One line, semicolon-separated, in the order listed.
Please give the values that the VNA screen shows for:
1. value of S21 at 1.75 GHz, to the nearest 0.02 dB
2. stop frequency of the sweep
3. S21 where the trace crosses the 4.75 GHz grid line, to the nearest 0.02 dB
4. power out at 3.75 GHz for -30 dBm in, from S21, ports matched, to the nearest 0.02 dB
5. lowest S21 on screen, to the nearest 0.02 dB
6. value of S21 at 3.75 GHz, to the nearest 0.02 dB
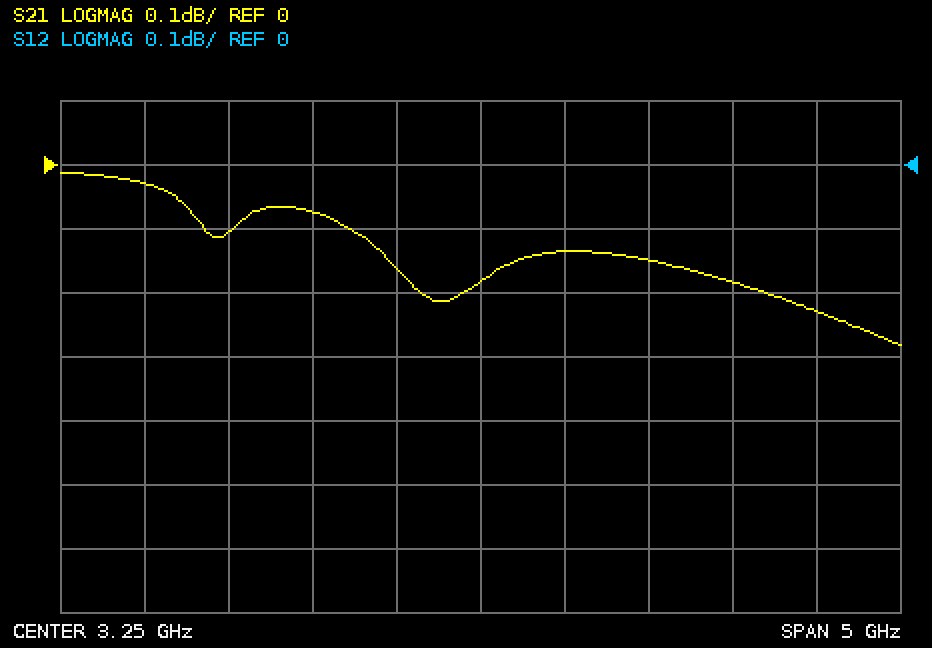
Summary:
-0.10 dB; 5.75 GHz; -0.18 dB; -30.14 dBm; -0.28 dB; -0.14 dB
